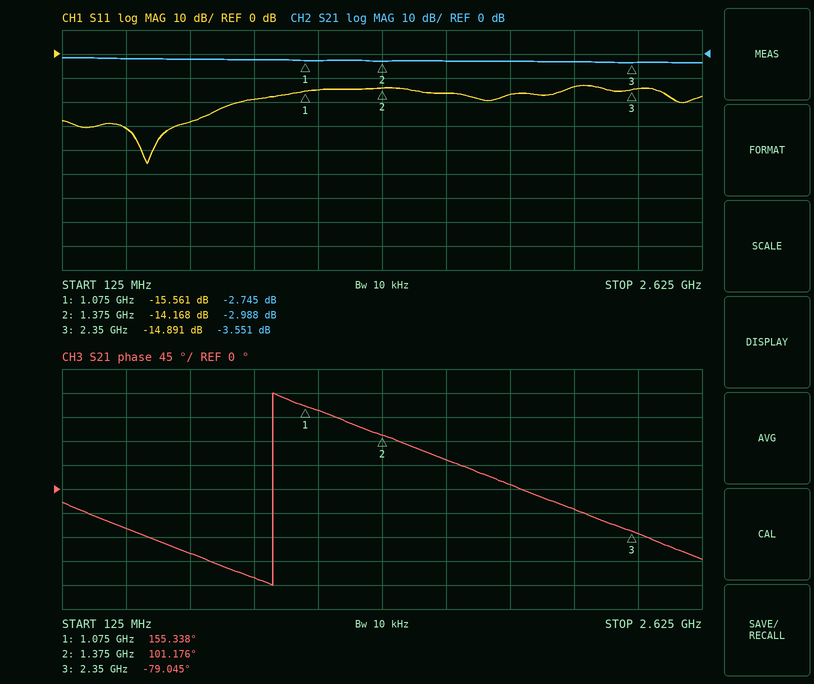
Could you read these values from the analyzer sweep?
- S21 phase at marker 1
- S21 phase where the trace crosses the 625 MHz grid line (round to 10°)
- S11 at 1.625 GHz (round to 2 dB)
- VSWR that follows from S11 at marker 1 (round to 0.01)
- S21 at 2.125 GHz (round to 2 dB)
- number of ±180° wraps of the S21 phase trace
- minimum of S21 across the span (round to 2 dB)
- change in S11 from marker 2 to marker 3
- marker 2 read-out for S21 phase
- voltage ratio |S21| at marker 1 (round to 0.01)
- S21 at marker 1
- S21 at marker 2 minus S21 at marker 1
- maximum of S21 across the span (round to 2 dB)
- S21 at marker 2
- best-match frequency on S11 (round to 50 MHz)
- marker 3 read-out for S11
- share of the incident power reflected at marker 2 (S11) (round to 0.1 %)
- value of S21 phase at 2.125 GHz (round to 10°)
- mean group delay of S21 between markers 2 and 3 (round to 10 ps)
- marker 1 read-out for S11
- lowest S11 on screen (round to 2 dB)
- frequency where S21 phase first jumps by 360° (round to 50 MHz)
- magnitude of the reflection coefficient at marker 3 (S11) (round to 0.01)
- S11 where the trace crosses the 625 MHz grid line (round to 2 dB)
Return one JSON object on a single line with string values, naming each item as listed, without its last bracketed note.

{"S21 phase at marker 1": "155.338°", "S21 phase where the trace crosses the 625 MHz grid line": "-120°", "S11 at 1.625 GHz": "-16 dB", "VSWR that follows from S11 at marker 1": "1.40", "S21 at 2.125 GHz": "-4 dB", "number of ±180° wraps of the S21 phase trace": "1", "minimum of S21 across the span": "-4 dB", "change in S11 from marker 2 to marker 3": "-0.723 dB", "marker 2 read-out for S21 phase": "101.176°", "voltage ratio |S21| at marker 1": "0.73", "S21 at marker 1": "-2.745 dB", "S21 at marker 2 minus S21 at marker 1": "-0.243 dB", "maximum of S21 across the span": "-2 dB", "S21 at marker 2": "-2.988 dB", "best-match frequency on S11": "450 MHz", "marker 3 read-out for S11": "-14.891 dB", "share of the incident power reflected at marker 2 (S11)": "3.8 %", "value of S21 phase at 2.125 GHz": "-40°", "mean group delay of S21 between markers 2 and 3": "510 ps", "marker 1 read-out for S11": "-15.561 dB", "lowest S11 on screen": "-46 dB", "frequency where S21 phase first jumps by 360°": "950 MHz", "magnitude of the reflection coefficient at marker 3 (S11)": "0.18", "S11 where the trace crosses the 625 MHz grid line": "-28 dB"}
